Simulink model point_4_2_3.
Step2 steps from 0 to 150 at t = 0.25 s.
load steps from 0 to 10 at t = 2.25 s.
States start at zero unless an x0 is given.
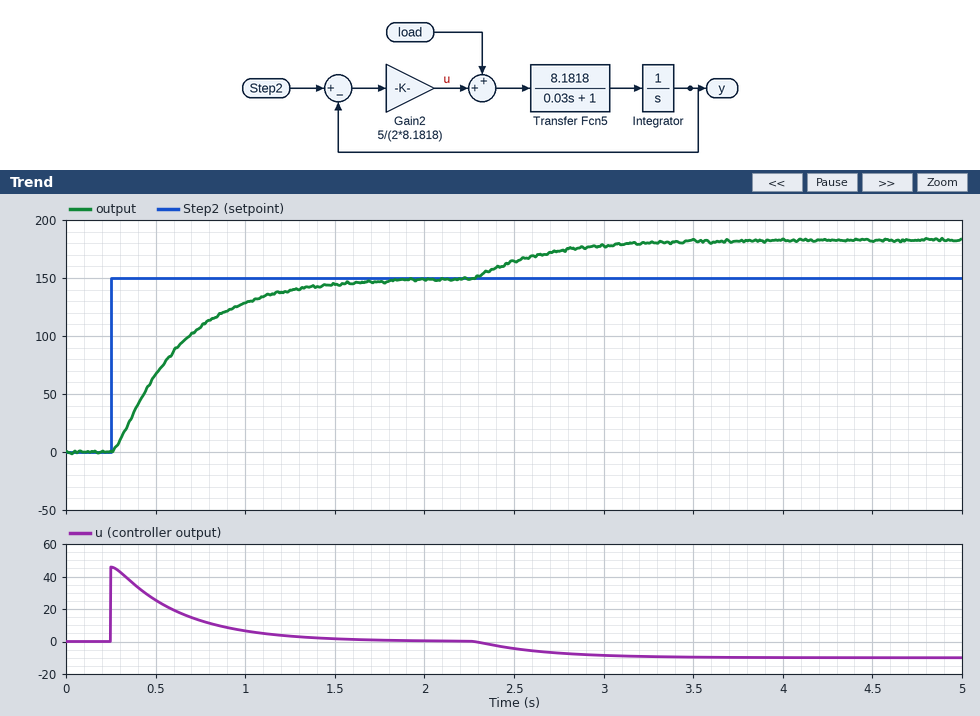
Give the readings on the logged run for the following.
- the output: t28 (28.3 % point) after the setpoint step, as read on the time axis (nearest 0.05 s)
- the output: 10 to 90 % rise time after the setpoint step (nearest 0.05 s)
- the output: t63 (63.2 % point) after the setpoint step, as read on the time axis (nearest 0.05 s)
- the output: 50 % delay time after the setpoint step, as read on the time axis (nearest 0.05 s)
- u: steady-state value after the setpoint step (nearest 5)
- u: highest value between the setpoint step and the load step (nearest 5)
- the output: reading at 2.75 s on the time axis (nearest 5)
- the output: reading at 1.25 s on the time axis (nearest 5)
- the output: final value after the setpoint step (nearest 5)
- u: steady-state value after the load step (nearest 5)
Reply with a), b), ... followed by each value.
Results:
a) 0.40 s
b) 0.80 s
c) 0.65 s
d) 0.55 s
e) 0
f) 45
g) 175
h) 140
i) 150
j) -10
